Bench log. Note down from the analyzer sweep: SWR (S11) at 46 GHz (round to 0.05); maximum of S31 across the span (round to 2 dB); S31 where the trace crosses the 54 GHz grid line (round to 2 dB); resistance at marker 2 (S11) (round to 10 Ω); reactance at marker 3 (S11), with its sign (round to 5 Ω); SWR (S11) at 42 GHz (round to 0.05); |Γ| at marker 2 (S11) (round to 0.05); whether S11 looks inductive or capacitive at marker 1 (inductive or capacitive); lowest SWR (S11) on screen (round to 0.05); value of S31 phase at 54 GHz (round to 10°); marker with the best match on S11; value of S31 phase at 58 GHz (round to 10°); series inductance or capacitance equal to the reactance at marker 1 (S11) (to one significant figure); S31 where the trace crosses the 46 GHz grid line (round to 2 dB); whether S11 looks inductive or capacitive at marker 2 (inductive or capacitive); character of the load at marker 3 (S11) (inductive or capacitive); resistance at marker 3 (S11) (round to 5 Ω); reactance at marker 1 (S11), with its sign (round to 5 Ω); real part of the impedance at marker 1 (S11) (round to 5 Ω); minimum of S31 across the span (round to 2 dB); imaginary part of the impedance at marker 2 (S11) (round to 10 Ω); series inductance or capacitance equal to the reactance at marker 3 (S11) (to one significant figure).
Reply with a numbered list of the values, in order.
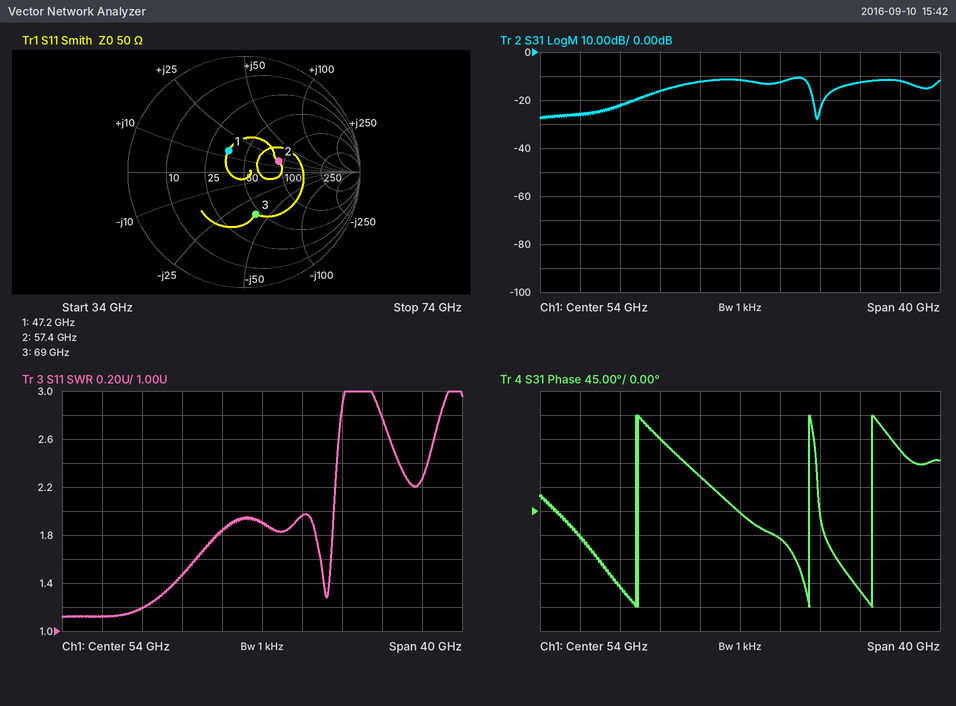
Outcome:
1. 1.45
2. -10 dB
3. -12 dB
4. 90 Ω
5. -40 Ω
6. 1.20
7. 0.30
8. inductive
9. 1.10
10. 0°
11. marker 1
12. -50°
13. 50 pH
14. -16 dB
15. inductive
16. capacitive
17. 45 Ω
18. +15 Ω
19. 35 Ω
20. -28 dB
21. +20 Ω
22. 60 fF
